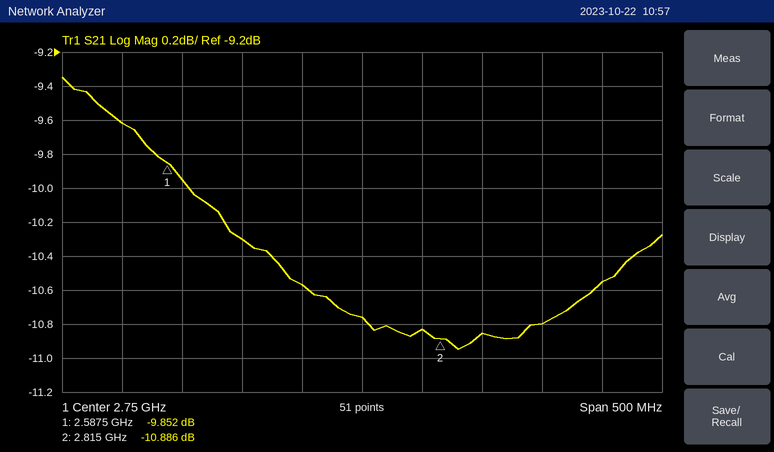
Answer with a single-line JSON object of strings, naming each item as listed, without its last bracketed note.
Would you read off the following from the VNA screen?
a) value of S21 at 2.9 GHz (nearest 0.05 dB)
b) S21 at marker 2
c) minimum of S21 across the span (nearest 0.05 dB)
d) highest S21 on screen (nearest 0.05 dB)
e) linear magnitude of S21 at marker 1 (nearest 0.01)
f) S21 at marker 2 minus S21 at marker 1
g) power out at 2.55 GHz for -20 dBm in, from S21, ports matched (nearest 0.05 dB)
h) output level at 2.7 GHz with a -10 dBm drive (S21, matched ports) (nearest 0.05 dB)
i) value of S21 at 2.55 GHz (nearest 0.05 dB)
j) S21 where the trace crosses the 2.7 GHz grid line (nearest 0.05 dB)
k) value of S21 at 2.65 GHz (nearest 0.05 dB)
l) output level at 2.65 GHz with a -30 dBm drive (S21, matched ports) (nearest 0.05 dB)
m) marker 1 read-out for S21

{"value of S21 at 2.9 GHz": "-10.80 dB", "S21 at marker 2": "-10.886 dB", "minimum of S21 across the span": "-10.95 dB", "highest S21 on screen": "-9.35 dB", "linear magnitude of S21 at marker 1": "0.32", "S21 at marker 2 minus S21 at marker 1": "-1.034 dB", "power out at 2.55 GHz for -20 dBm in, from S21, ports matched": "-29.60 dBm", "output level at 2.7 GHz with a -10 dBm drive (S21, matched ports)": "-20.55 dBm", "value of S21 at 2.55 GHz": "-9.60 dB", "S21 where the trace crosses the 2.7 GHz grid line": "-10.55 dB", "value of S21 at 2.65 GHz": "-10.30 dB", "output level at 2.65 GHz with a -30 dBm drive (S21, matched ports)": "-40.30 dBm", "marker 1 read-out for S21": "-9.852 dB"}
